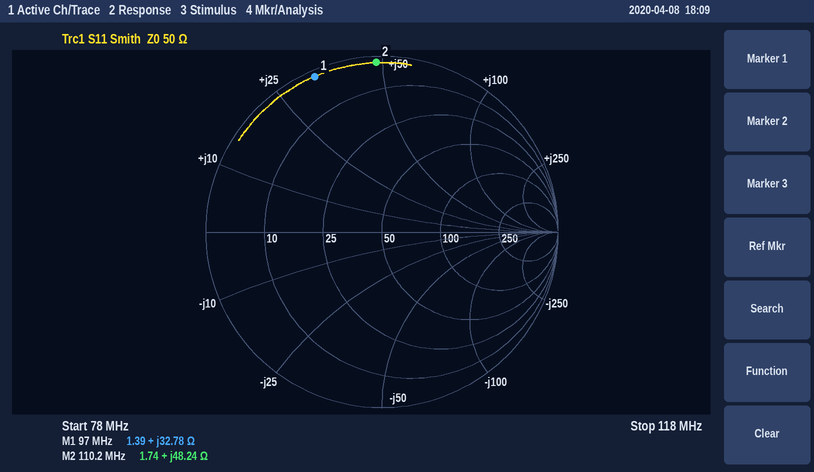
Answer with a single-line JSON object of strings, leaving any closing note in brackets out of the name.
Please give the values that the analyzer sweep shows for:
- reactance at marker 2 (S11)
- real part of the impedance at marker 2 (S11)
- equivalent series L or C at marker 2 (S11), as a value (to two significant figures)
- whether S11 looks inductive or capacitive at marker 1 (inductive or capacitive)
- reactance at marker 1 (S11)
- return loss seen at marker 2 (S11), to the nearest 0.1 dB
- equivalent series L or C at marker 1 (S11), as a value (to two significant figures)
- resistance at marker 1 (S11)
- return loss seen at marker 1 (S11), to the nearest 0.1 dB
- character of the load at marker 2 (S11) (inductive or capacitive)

{"reactance at marker 2": "+48.24 Ω", "real part of the impedance at marker 2": "1.74 Ω", "equivalent series L or C at marker 2 (S11), as a value": "70 nH", "whether S11 looks inductive or capacitive at marker 1": "inductive", "reactance at marker 1": "+32.78 Ω", "return loss seen at marker 2 (S11), to the nearest 0.1 dB": "0.3 dB", "equivalent series L or C at marker 1 (S11), as a value": "54 nH", "resistance at marker 1": "1.39 Ω", "return loss seen at marker 1 (S11), to the nearest 0.1 dB": "0.3 dB", "character of the load at marker 2 (S11)": "inductive"}
